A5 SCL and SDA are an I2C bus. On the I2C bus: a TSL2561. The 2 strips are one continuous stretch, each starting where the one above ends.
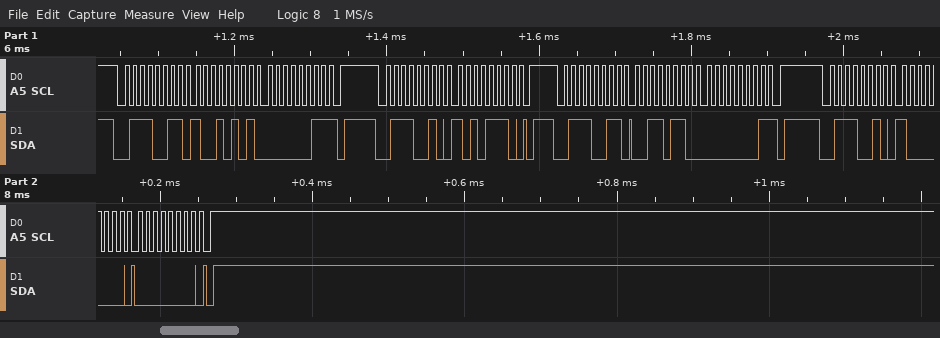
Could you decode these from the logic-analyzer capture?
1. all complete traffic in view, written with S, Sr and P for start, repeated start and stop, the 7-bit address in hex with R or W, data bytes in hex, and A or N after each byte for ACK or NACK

S 39R A 95 A 03 N P S 39W A AE A P S 39R A 36 A 01 N P S 39W A 80 A 00 A P
